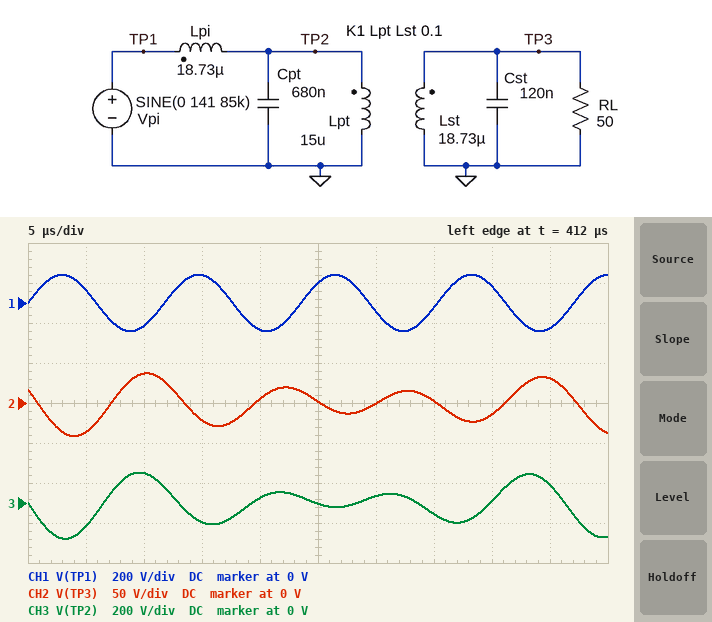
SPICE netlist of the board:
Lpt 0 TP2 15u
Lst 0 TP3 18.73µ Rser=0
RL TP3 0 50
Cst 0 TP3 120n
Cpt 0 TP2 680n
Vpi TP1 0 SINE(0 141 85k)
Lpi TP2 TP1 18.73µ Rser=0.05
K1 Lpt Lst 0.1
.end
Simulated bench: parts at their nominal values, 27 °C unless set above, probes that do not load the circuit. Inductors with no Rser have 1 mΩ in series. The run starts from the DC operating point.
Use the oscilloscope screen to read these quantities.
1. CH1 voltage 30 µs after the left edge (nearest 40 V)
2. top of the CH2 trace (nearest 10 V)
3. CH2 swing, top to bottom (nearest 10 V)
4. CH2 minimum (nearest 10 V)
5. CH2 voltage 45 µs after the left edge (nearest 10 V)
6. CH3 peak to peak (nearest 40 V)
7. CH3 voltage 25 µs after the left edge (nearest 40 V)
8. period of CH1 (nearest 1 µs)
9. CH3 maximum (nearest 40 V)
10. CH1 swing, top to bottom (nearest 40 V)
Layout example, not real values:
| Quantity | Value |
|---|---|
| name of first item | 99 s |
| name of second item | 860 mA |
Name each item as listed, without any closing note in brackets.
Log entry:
| Quantity | Value |
|---|---|
| CH1 voltage 30 µs after the left edge | -40 V |
| top of the CH2 trace | 40 V |
| CH2 swing, top to bottom | 80 V |
| CH2 minimum | -40 V |
| CH2 voltage 45 µs after the left edge | 30 V |
| CH3 peak to peak | 320 V |
| CH3 voltage 25 µs after the left edge | 0 V |
| period of CH1 | 12 µs |
| CH3 maximum | 160 V |
| CH1 swing, top to bottom | 280 V |
